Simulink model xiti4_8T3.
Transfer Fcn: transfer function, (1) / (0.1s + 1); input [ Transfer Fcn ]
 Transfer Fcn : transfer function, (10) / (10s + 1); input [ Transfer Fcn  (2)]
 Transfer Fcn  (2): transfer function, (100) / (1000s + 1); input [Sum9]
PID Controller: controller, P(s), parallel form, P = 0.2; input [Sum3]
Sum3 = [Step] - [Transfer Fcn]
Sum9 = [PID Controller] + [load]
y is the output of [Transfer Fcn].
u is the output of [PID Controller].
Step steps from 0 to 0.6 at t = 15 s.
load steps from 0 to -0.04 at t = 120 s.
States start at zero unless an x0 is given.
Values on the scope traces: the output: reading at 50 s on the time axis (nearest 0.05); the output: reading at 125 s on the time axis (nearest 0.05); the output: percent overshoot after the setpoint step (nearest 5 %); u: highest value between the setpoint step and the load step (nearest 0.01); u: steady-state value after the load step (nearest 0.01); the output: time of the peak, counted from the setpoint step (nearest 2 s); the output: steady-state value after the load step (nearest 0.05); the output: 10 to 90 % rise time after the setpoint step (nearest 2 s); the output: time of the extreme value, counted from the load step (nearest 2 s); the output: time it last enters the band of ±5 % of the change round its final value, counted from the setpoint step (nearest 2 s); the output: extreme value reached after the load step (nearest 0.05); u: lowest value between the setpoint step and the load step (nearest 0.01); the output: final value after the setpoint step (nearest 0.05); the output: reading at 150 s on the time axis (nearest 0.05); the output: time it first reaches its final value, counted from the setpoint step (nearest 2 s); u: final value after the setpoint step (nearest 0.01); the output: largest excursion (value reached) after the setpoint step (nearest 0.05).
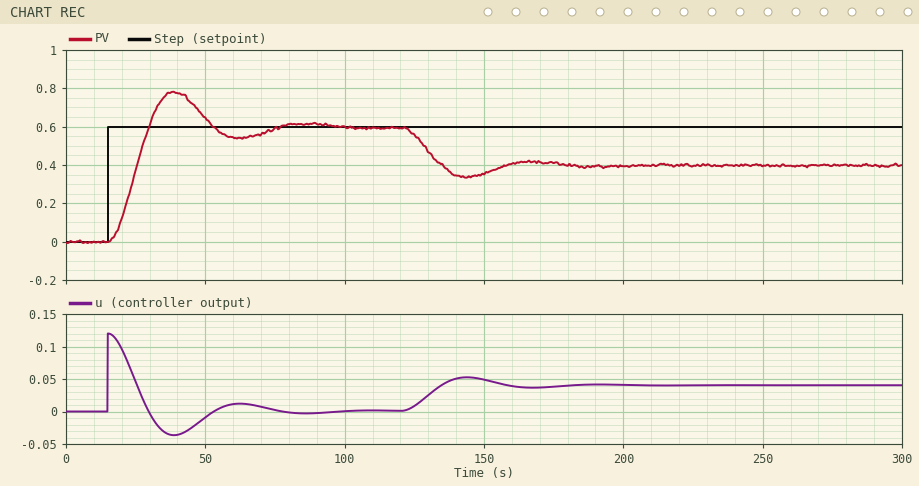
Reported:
0.65
0.55
30 %
0.12
0.04
24 s
0.40
10 s
24 s
56 s
0.35
-0.04
0.60
0.35
14 s
0.00
0.80
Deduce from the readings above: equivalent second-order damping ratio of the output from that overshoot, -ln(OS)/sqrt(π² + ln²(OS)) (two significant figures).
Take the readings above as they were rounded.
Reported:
0.36
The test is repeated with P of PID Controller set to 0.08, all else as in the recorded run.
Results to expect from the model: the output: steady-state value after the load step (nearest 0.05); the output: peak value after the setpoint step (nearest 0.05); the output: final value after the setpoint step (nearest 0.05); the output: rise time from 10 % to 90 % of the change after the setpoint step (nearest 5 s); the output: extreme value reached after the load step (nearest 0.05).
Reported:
0.10
0.65
0.60
20 s
0.05
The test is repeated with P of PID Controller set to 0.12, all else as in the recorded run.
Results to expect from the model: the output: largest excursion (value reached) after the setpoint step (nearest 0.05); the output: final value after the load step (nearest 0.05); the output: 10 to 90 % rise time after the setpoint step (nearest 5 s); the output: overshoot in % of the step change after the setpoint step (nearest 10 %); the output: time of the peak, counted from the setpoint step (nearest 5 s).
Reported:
0.70
0.25
15 s
20 %
30 s
